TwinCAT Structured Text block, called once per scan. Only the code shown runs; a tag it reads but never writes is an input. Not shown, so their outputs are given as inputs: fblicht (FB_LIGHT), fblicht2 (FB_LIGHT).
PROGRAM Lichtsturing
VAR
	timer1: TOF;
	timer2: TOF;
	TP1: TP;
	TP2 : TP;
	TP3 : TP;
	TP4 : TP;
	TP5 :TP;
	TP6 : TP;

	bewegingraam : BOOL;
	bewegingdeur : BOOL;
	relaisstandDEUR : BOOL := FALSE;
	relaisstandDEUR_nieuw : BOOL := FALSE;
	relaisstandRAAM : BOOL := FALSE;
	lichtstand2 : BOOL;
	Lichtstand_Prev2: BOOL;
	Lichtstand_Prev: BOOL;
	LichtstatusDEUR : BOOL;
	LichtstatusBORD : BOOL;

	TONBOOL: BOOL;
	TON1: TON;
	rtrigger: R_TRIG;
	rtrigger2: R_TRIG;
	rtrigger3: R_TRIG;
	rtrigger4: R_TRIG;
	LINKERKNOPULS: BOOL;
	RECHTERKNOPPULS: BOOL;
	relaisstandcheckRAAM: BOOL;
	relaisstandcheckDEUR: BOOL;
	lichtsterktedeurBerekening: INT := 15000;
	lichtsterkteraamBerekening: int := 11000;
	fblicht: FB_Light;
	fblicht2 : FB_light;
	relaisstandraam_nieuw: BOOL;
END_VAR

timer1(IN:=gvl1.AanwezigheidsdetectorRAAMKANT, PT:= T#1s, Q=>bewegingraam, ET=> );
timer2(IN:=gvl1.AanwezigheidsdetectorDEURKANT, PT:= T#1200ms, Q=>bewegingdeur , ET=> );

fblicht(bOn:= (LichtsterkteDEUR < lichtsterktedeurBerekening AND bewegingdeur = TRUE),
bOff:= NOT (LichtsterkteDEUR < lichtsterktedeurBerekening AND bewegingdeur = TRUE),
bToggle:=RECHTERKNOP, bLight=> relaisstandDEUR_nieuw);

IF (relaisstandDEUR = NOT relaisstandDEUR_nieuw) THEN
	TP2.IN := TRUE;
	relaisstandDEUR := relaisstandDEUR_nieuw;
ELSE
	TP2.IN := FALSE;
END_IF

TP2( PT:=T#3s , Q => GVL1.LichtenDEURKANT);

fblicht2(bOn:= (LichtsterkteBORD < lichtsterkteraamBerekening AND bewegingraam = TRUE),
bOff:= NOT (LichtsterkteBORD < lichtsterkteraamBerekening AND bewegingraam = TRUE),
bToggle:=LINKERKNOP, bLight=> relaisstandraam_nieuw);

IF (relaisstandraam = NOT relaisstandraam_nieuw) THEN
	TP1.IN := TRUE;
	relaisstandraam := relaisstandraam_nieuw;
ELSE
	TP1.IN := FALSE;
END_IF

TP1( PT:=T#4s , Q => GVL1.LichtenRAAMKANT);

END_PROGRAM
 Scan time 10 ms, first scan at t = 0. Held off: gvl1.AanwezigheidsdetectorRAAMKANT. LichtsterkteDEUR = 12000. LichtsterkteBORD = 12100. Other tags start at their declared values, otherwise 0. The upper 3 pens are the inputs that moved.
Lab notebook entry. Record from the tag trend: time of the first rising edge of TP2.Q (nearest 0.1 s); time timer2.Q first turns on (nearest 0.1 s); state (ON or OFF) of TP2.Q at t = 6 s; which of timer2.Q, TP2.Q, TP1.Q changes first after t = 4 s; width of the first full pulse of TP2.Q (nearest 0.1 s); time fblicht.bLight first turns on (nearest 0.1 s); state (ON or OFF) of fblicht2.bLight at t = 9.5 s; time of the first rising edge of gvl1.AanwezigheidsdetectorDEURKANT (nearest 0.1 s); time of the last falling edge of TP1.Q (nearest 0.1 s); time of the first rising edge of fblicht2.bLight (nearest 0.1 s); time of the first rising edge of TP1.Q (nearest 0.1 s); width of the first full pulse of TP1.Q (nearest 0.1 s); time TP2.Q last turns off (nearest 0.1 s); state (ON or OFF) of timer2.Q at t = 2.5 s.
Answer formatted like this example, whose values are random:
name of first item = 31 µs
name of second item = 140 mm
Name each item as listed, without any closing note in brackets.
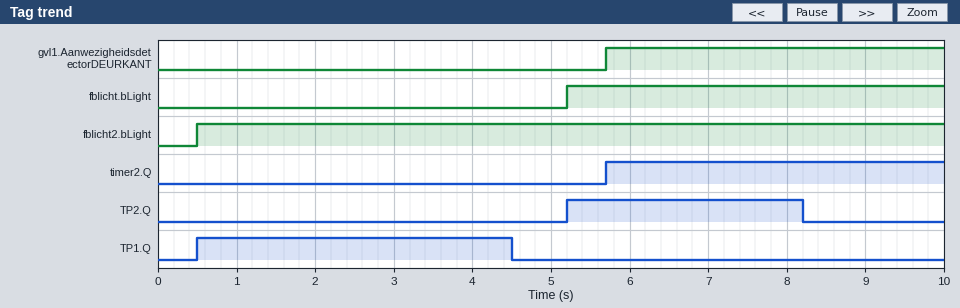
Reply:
time of the first rising edge of TP2.Q = 5.2 s
time timer2.Q first turns on = 5.7 s
state (ON or OFF) of TP2.Q at t = 6 s = ON
which of timer2.Q, TP2.Q, TP1.Q changes first after t = 4 s = TP1.Q
width of the first full pulse of TP2.Q = 3.0 s
time fblicht.bLight first turns on = 5.2 s
state (ON or OFF) of fblicht2.bLight at t = 9.5 s = ON
time of the first rising edge of gvl1.AanwezigheidsdetectorDEURKANT = 5.7 s
time of the last falling edge of TP1.Q = 4.5 s
time of the first rising edge of fblicht2.bLight = 0.5 s
time of the first rising edge of TP1.Q = 0.5 s
width of the first full pulse of TP1.Q = 4.0 s
time TP2.Q last turns off = 8.2 s
state (ON or OFF) of timer2.Q at t = 2.5 s = OFF
